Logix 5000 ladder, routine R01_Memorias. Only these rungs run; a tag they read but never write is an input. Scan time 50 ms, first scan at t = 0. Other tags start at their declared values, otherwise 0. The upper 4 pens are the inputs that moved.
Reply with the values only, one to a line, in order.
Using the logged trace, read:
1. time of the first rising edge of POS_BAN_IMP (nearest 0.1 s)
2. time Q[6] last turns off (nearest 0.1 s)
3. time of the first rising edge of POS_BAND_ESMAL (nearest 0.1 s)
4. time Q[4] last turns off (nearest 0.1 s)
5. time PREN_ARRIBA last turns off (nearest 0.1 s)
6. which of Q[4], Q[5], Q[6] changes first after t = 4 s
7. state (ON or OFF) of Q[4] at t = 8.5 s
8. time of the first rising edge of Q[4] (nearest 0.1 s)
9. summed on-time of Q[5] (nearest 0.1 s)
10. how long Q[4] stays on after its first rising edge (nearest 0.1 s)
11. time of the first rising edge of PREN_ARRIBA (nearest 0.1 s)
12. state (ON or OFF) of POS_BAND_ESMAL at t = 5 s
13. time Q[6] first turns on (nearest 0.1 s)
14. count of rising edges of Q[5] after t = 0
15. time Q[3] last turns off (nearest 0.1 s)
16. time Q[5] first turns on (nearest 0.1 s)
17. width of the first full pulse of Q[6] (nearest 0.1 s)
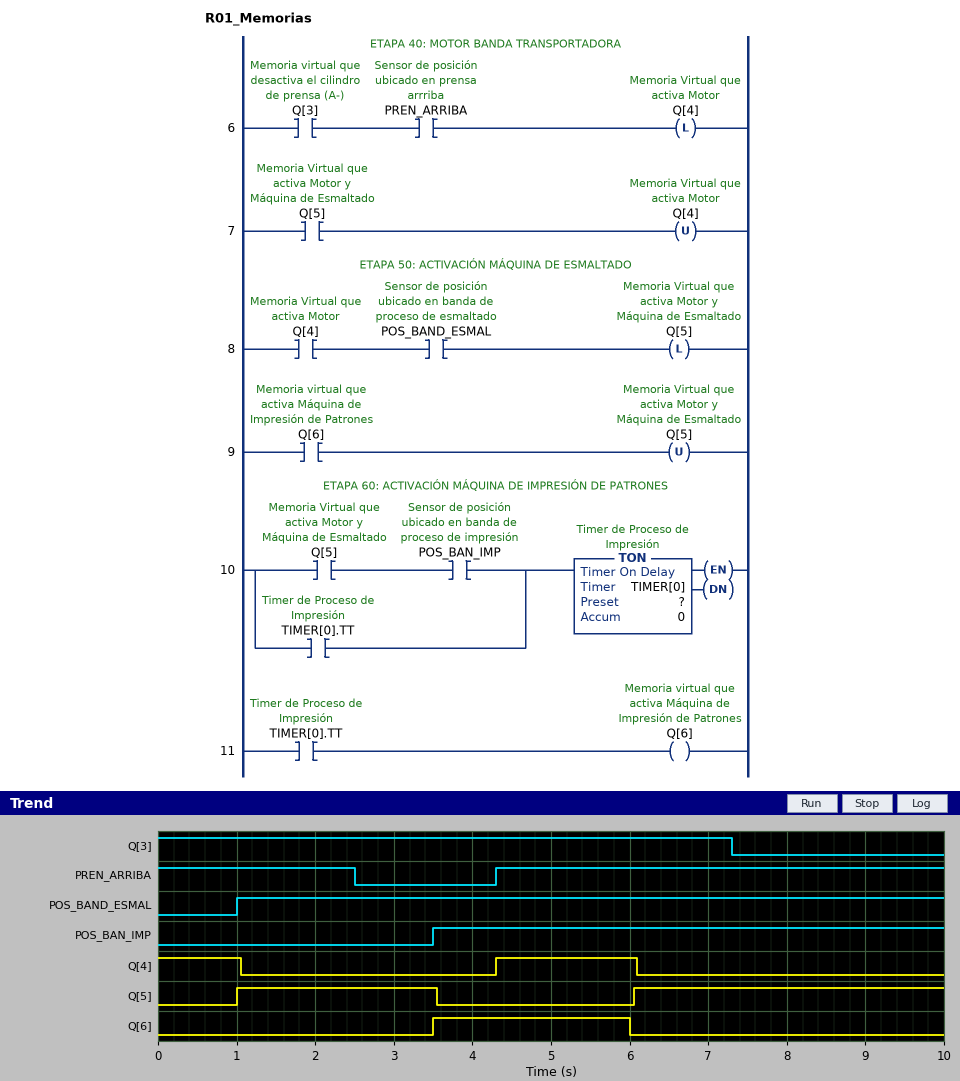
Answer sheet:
3.5 s
6.0 s
1.0 s
6.1 s
2.5 s
Q[4]
OFF
4.3 s
6.5 s
1.8 s
4.3 s
ON
3.5 s
2
7.3 s
1.0 s
2.5 s
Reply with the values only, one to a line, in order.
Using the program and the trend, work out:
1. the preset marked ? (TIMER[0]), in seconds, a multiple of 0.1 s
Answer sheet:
2.5 s
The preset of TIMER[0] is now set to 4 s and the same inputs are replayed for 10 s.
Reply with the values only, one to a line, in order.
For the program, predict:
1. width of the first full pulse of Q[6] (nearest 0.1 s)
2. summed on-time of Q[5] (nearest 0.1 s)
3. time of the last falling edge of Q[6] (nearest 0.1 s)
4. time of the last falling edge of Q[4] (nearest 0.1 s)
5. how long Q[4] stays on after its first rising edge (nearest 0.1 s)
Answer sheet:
4.0 s
5.0 s
7.5 s
7.6 s
3.3 s
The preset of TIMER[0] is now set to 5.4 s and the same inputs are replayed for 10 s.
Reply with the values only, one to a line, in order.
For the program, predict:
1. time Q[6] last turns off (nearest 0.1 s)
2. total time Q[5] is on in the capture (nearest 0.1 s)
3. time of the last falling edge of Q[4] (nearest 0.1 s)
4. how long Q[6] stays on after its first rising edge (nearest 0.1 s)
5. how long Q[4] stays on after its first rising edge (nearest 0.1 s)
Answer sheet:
8.9 s
3.6 s
9.0 s
5.4 s
4.7 s
